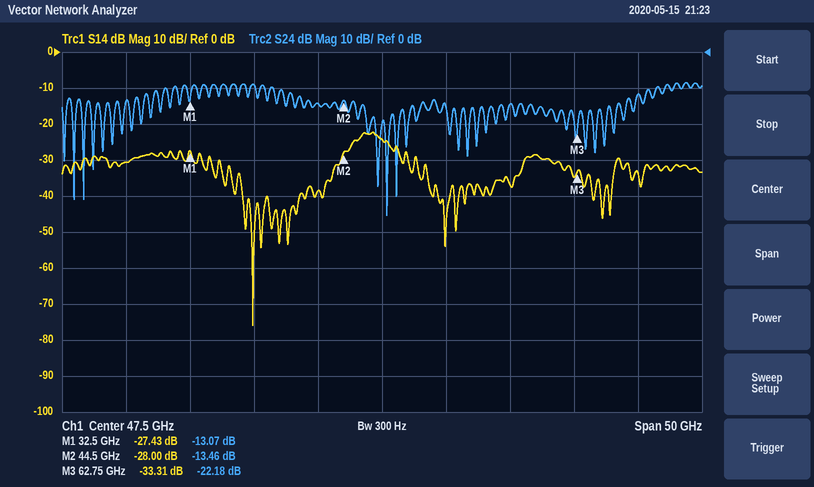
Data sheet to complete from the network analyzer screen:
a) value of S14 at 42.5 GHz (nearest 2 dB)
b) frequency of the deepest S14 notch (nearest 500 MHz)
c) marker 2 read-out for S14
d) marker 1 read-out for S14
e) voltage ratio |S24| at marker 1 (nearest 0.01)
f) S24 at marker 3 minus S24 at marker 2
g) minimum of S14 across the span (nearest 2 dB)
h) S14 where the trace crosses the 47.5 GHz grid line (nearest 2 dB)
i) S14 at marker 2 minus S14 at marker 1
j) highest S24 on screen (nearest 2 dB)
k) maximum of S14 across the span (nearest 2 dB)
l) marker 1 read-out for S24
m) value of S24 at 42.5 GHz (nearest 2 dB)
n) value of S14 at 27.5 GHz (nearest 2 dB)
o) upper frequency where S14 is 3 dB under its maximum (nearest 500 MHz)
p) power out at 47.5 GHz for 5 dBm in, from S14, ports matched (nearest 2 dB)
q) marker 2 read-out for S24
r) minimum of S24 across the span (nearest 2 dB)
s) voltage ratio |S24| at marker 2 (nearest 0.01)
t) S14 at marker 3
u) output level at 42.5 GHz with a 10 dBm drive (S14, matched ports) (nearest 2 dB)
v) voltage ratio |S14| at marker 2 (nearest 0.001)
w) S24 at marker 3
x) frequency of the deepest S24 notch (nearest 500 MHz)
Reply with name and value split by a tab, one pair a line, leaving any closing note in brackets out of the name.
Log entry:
value of S14 at 42.5 GHz	-38 dB
frequency of the deepest S14 notch	37.5 GHz
marker 2 read-out for S14	-28.00 dB
marker 1 read-out for S14	-27.43 dB
voltage ratio |S24| at marker 1	0.22
S24 at marker 3 minus S24 at marker 2	-8.72 dB
minimum of S14 across the span	-76 dB
S14 where the trace crosses the 47.5 GHz grid line	-24 dB
S14 at marker 2 minus S14 at marker 1	-0.57 dB
highest S24 on screen	-8 dB
maximum of S14 across the span	-22 dB
marker 1 read-out for S24	-13.07 dB
value of S24 at 42.5 GHz	-14 dB
value of S14 at 27.5 GHz	-30 dB
upper frequency where S14 is 3 dB under its maximum	48.0 GHz
power out at 47.5 GHz for 5 dBm in, from S14, ports matched	-20 dBm
marker 2 read-out for S24	-13.46 dB
minimum of S24 across the span	-46 dB
voltage ratio |S24| at marker 2	0.21
S14 at marker 3	-33.31 dB
output level at 42.5 GHz with a 10 dBm drive (S14, matched ports)	-28 dBm
voltage ratio |S14| at marker 2	0.040
S24 at marker 3	-22.18 dB
frequency of the deepest S24 notch	48.0 GHz
